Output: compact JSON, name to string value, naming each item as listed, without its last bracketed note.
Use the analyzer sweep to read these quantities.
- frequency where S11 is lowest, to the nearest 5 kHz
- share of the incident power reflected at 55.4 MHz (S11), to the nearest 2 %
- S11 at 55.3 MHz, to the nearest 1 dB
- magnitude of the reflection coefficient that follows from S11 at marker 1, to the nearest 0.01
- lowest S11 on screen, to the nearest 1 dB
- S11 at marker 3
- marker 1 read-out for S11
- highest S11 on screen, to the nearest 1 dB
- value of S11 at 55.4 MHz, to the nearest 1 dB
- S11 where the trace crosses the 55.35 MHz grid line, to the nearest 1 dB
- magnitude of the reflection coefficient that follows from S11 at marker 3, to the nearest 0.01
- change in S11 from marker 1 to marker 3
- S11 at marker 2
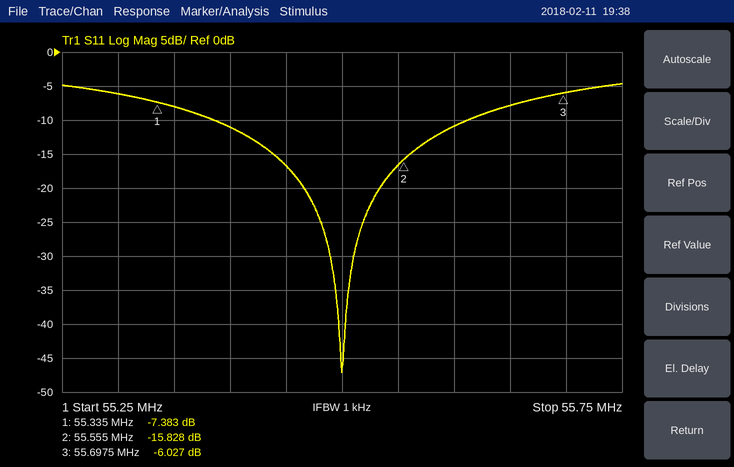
{"frequency where S11 is lowest, to the nearest 5 kHz": "55.500 MHz", "share of the incident power reflected at 55.4 MHz (S11), to the nearest 2 %": "8 %", "S11 at 55.3 MHz, to the nearest 1 dB": "-6 dB", "magnitude of the reflection coefficient that follows from S11 at marker 1, to the nearest 0.01": "0.43", "lowest S11 on screen, to the nearest 1 dB": "-47 dB", "S11 at marker 3": "-6.027 dB", "marker 1 read-out for S11": "-7.383 dB", "highest S11 on screen, to the nearest 1 dB": "-5 dB", "value of S11 at 55.4 MHz, to the nearest 1 dB": "-11 dB", "S11 where the trace crosses the 55.35 MHz grid line, to the nearest 1 dB": "-8 dB", "magnitude of the reflection coefficient that follows from S11 at marker 3, to the nearest 0.01": "0.50", "change in S11 from marker 1 to marker 3": "1.356 dB", "S11 at marker 2": "-15.828 dB"}
